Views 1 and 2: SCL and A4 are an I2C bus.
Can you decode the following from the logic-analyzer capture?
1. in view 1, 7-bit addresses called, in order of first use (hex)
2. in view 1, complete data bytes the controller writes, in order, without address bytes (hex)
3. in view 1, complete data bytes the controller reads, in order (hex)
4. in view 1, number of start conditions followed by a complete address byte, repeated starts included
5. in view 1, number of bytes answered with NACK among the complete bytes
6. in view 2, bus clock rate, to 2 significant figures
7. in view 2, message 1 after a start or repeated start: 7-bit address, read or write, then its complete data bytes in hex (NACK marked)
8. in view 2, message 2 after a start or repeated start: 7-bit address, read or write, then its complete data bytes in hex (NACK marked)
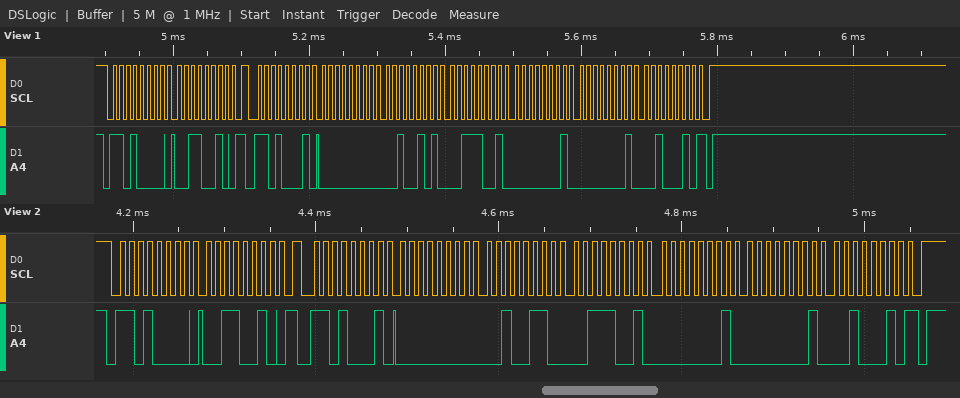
0x68
32
00 25 39 01 01 22
2
1
100 kHz
0x68 write: 32
0x68 read: 00 26 39 01 01 22 NACK
